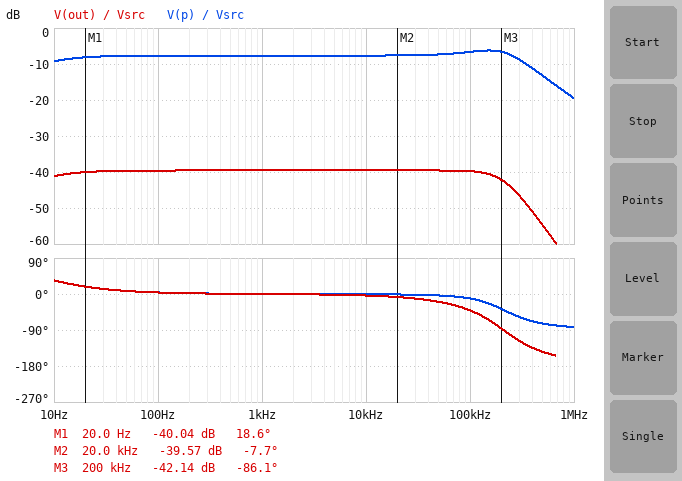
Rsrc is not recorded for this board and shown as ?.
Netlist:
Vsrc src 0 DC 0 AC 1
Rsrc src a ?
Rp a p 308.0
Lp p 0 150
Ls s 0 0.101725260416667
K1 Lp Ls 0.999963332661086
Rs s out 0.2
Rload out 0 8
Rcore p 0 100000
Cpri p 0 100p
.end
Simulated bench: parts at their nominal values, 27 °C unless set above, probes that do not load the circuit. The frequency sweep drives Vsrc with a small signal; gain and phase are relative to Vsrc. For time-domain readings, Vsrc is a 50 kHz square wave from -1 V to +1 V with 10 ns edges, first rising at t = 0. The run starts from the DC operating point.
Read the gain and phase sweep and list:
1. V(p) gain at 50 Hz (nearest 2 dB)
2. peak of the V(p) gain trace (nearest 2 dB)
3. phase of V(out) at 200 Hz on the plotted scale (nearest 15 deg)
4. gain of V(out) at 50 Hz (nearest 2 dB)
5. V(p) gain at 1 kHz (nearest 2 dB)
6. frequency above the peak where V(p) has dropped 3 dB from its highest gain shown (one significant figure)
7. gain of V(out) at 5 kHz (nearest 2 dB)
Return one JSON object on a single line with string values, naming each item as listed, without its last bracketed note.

{"V(p) gain at 50 Hz": "-8 dB", "peak of the V(p) gain trace": "-6 dB", "phase of V(out) at 200 Hz on the plotted scale": "0 deg", "gain of V(out) at 50 Hz": "-40 dB", "V(p) gain at 1 kHz": "-8 dB", "frequency above the peak where V(p) has dropped 3 dB from its highest gain shown": "300 kHz", "gain of V(out) at 5 kHz": "-40 dB"}
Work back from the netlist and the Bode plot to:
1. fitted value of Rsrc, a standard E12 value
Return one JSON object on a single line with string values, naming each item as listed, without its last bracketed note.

{"fitted value of Rsrc, a standard E12 value": "15 kΩ"}
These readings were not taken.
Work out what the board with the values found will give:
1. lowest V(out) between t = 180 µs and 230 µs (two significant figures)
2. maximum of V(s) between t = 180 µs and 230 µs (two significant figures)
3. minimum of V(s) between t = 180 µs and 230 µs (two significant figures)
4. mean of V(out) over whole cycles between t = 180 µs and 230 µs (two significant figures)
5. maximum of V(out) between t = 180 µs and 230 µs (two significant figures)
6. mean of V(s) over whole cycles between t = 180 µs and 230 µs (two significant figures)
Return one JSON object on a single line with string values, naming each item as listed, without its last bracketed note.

{"lowest V(out) between t = 180 µs and 230 µs": "-1.0 mV", "maximum of V(s) between t = 180 µs and 230 µs": "22 mV", "minimum of V(s) between t = 180 µs and 230 µs": "-1.1 mV", "mean of V(out) over whole cycles between t = 180 µs and 230 µs": "10 mV", "maximum of V(out) between t = 180 µs and 230 µs": "22 mV", "mean of V(s) over whole cycles between t = 180 µs and 230 µs": "11 mV"}
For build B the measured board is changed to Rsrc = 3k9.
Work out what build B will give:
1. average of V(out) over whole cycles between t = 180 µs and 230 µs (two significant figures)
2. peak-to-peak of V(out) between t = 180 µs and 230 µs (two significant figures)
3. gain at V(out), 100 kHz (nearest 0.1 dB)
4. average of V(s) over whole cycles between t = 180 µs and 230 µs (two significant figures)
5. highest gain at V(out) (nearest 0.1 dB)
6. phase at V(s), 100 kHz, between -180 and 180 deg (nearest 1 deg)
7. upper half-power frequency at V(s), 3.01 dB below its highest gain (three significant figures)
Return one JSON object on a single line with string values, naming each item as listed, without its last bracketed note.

{"average of V(out) over whole cycles between t = 180 µs and 230 µs": "18 mV", "peak-to-peak of V(out) between t = 180 µs and 230 µs": "37 mV", "gain at V(out), 100 kHz": "-35.5 dB", "average of V(s) over whole cycles between t = 180 µs and 230 µs": "19 mV", "highest gain at V(out)": "-34.8 dB", "phase at V(s), 100 kHz, between -180 and 180 deg": "-35 deg", "upper half-power frequency at V(s), 3.01 dB below its highest gain": "214 kHz"}
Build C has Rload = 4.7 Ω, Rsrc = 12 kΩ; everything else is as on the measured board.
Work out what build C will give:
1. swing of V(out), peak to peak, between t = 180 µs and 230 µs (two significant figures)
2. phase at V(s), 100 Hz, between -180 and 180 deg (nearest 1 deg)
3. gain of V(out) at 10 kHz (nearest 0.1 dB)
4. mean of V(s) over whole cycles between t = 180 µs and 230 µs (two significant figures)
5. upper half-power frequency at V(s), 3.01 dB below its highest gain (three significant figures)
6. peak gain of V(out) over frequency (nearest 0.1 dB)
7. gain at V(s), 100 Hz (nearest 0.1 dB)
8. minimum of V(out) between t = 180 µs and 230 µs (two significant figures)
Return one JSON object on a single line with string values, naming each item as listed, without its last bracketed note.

{"swing of V(out), peak to peak, between t = 180 µs and 230 µs": "20 mV", "phase at V(s), 100 Hz, between -180 and 180 deg": "3 deg", "gain of V(out) at 10 kHz": "-41.1 dB", "mean of V(s) over whole cycles between t = 180 µs and 230 µs": "9.2 mV", "upper half-power frequency at V(s), 3.01 dB below its highest gain": "211 kHz", "peak gain of V(out) over frequency": "-40.9 dB", "gain at V(s), 100 Hz": "-40.7 dB", "minimum of V(out) between t = 180 µs and 230 µs": "-1.4 mV"}
